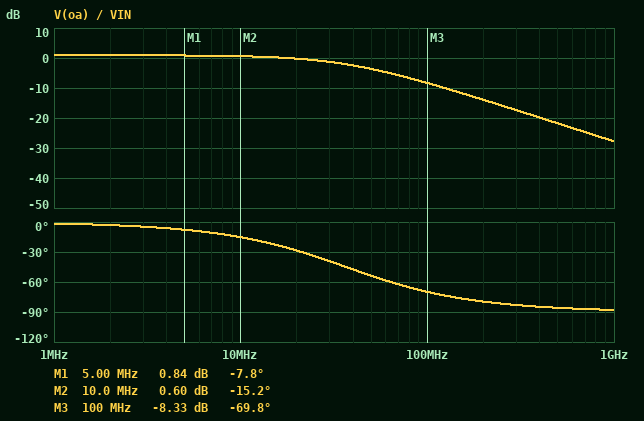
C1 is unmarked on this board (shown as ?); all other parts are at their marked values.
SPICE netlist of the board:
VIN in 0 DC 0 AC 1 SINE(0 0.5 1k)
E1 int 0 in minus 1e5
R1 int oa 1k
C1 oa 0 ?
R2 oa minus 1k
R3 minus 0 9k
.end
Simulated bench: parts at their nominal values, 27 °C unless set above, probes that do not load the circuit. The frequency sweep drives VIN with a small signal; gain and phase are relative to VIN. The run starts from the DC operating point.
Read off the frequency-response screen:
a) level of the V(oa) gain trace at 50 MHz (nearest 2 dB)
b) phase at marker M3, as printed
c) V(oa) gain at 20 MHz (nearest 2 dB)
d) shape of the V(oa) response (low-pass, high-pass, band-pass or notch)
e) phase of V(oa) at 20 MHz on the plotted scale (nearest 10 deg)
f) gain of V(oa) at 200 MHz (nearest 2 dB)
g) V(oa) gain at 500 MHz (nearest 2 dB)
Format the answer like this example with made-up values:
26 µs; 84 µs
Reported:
-4 dB; -69.8 deg; 0 dB; low-pass; -30 deg; -14 dB; -22 dB
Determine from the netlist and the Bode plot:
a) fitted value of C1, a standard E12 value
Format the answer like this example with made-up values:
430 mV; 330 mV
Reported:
390 nF
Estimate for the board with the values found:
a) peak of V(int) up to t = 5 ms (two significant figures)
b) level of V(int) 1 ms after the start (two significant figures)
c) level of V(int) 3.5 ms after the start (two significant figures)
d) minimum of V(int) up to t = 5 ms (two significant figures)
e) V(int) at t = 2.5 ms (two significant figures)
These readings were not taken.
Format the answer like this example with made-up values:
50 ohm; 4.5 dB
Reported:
1.5 V; 1.4 V; -1.4 V; -1.5 V; -1.4 V
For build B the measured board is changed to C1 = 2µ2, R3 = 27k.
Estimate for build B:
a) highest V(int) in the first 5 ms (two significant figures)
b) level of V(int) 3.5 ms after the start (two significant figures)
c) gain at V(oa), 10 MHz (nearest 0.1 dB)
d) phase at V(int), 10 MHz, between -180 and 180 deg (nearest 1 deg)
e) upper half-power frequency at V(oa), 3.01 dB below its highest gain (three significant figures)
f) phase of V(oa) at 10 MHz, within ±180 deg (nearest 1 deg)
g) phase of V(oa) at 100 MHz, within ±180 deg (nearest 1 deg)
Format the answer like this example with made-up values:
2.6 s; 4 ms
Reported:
7.2 V; -7.2 V; -4.5 dB; 35 deg; 6.98 MHz; -55 deg; -86 deg
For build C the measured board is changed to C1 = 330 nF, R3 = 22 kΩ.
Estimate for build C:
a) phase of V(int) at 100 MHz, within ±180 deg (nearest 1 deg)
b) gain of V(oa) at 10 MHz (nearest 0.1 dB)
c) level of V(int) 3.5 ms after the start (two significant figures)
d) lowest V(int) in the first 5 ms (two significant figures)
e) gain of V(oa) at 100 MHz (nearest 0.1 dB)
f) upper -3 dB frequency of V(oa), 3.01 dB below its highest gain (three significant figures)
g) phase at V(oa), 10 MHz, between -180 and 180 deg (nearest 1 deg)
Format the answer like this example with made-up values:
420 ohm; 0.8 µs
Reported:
25 deg; 0.2 dB; -1.1 V; -1.2 V; -7.2 dB; 46.1 MHz; -12 deg
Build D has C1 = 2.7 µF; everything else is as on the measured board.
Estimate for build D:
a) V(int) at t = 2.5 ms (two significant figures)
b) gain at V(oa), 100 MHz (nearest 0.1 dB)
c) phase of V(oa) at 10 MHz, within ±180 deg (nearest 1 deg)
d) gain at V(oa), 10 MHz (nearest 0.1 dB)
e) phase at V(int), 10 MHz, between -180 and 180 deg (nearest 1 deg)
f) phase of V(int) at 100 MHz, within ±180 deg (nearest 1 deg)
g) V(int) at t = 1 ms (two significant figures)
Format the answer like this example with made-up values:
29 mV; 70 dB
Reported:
-9.4 V; -24.6 dB; -62 deg; -5.7 dB; 28 deg; 3 deg; 9.4 V
